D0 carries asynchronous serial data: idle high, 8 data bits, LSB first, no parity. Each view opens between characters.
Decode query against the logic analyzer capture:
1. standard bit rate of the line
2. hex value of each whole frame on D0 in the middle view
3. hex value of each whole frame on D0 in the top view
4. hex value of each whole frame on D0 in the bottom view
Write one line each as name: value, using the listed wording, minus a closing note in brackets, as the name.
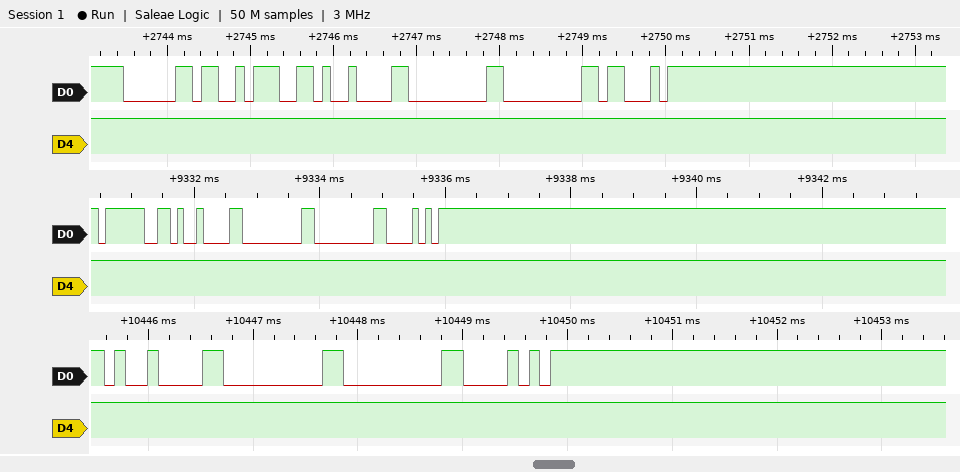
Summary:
standard bit rate of the line: 9600 baud
hex value of each whole frame on D0 in the middle view: 3F, 09, 00, 00, A8
hex value of each whole frame on D0 in the top view: 60, 3A, 09, 00, 00, A3
hex value of each whole frame on D0 in the bottom view: 09, 00, 00, A8
